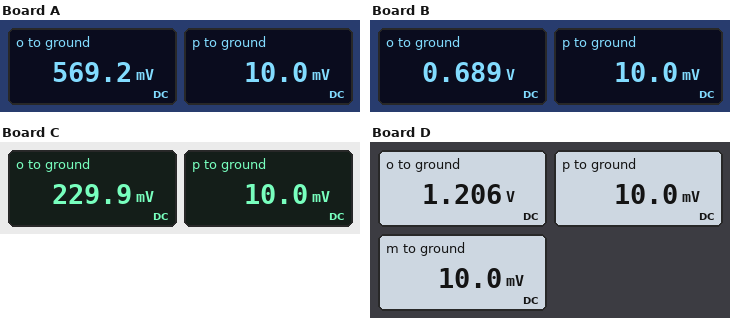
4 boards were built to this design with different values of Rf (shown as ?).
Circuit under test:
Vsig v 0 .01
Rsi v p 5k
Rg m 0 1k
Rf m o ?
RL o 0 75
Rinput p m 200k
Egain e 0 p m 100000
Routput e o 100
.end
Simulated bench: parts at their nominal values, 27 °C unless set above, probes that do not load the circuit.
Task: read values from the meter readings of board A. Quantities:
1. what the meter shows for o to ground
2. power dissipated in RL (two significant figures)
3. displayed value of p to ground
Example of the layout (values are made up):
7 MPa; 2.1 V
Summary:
569.2 mV; 4.3 mW; 10.0 mV
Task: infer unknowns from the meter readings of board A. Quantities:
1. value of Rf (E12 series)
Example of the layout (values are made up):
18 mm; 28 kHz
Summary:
56 kΩ
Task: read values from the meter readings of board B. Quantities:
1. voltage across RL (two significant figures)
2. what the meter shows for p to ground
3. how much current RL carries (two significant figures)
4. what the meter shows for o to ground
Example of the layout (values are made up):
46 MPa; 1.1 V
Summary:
690 mV; 10.0 mV; 9.2 mA; 0.689 V
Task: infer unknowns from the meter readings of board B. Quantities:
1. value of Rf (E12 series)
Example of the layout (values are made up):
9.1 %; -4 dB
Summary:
68 kΩ
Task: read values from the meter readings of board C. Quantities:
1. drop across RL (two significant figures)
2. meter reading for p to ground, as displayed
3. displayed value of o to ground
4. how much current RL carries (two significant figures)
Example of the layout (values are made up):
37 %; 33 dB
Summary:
230 mV; 10.0 mV; 229.9 mV; 3.1 mA
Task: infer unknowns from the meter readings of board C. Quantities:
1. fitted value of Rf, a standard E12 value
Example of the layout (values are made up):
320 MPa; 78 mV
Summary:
22 kΩ
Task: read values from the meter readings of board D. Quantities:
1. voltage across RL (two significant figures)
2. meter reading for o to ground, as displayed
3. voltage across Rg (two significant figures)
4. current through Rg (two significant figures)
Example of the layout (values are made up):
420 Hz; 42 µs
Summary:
1.2 V; 1.206 V; 10 mV; 10 µA
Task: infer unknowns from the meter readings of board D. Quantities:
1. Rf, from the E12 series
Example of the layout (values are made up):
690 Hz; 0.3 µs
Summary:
120 kΩ
